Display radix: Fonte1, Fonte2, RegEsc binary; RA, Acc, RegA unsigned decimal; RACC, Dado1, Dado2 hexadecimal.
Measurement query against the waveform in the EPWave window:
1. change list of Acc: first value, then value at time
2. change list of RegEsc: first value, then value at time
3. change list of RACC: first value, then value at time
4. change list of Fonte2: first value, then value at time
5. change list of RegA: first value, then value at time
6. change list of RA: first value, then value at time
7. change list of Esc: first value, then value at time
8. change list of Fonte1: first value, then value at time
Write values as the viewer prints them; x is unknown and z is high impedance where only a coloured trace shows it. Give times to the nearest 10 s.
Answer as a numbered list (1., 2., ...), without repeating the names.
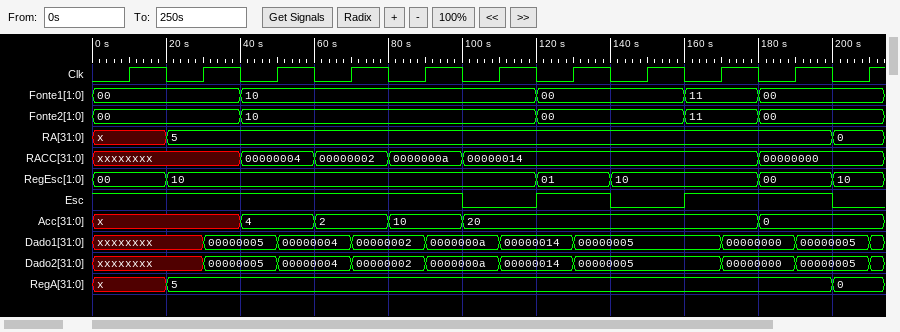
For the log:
1. x, 4 at 40 s, 2 at 60 s, 10 at 80 s, 20 at 100 s, 0 at 180 s
2. 00, 10 at 20 s, 01 at 120 s, 10 at 140 s, 00 at 180 s, 10 at 200 s
3. xxxxxxxx, 00000004 at 40 s, 00000002 at 60 s, 0000000a at 80 s, 00000014 at 100 s, 00000000 at 180 s
4. 00, 10 at 40 s, 00 at 120 s, 11 at 160 s, 00 at 180 s
5. x, 5 at 20 s, 0 at 200 s
6. x, 5 at 20 s, 0 at 200 s
7. 1, 0 at 100 s, 1 at 120 s, 0 at 140 s, 1 at 160 s, 0 at 200 s
8. 00, 10 at 40 s, 00 at 120 s, 11 at 160 s, 00 at 180 s
